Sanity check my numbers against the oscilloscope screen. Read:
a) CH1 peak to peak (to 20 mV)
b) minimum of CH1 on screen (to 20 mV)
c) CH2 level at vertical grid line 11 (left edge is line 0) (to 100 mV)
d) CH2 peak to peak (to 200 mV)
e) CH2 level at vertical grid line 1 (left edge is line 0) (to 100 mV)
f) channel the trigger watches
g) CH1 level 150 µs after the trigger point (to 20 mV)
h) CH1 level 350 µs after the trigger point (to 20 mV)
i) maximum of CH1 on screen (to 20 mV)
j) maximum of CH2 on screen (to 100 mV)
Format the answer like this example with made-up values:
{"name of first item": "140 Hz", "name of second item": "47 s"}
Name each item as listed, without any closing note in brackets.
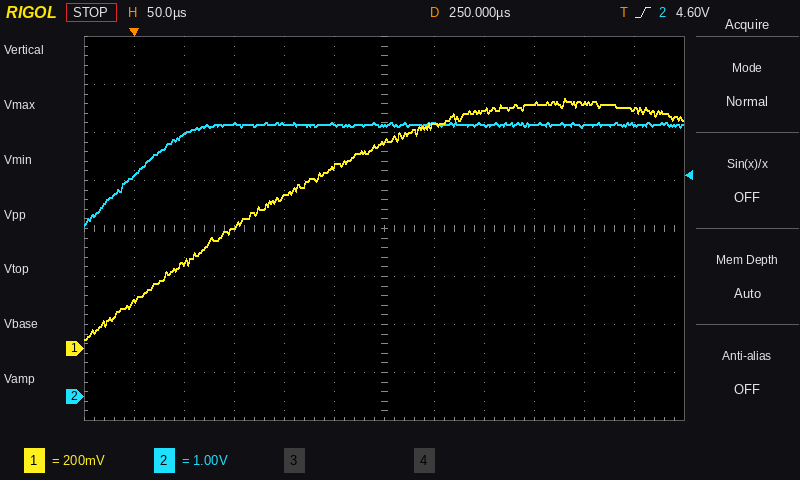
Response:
{"CH1 peak to peak": "1.00 V", "minimum of CH1 on screen": "40 mV", "CH2 level at vertical grid line 11 (left edge is line 0)": "5.7 V", "CH2 peak to peak": "2.2 V", "CH2 level at vertical grid line 1 (left edge is line 0)": "4.6 V", "channel the trigger watches": "CH2", "CH1 level 150 µs after the trigger point": "640 mV", "CH1 level 350 µs after the trigger point": "1.00 V", "maximum of CH1 on screen": "1.04 V", "maximum of CH2 on screen": "5.7 V"}
